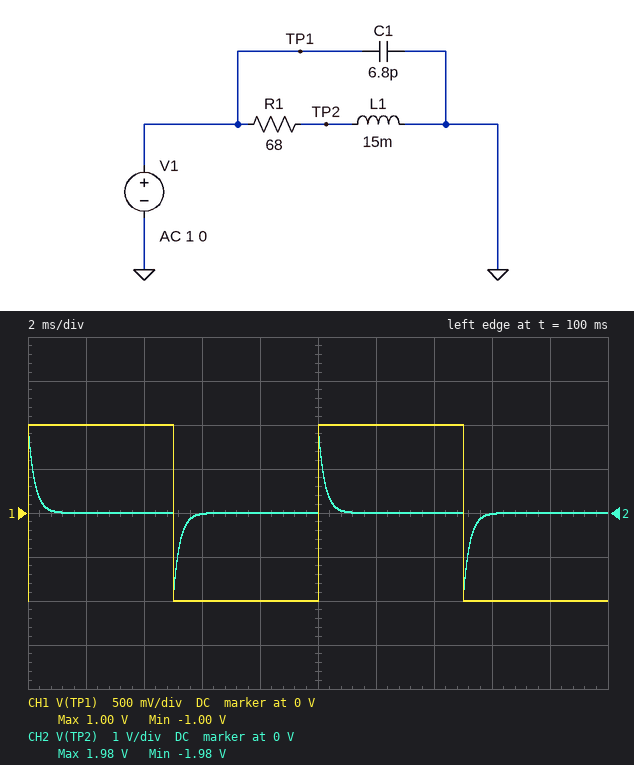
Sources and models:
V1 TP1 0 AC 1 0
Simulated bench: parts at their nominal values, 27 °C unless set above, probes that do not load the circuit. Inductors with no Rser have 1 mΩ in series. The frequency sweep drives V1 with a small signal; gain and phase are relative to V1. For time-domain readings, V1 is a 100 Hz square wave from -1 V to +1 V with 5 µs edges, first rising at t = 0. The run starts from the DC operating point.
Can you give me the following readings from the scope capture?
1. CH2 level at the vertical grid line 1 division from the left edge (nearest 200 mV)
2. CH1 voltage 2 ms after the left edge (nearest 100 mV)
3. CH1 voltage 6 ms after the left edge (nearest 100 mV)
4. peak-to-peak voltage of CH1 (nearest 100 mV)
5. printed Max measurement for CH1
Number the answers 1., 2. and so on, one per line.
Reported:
1. 0 V
2. 1.0 V
3. -1.0 V
4. 2.0 V
5. 1.00 V
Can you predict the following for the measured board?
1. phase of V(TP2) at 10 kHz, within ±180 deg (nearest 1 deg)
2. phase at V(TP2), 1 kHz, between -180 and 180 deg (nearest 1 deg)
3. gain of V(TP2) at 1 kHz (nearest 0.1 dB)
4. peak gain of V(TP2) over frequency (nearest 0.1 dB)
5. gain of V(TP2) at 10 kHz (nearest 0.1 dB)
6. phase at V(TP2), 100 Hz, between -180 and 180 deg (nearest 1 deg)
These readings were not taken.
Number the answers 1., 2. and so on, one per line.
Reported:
1. 4 deg
2. 36 deg
3. -1.8 dB
4. 0 dB
5. 0 dB
6. 82 deg
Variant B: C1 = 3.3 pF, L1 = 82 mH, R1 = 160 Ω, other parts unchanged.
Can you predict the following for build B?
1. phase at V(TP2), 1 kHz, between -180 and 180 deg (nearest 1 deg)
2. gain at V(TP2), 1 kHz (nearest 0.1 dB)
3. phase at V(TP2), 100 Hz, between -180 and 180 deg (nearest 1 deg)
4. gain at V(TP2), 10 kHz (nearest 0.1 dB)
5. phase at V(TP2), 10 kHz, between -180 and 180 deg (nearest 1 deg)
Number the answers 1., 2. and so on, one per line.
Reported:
1. 17 deg
2. -0.4 dB
3. 72 deg
4. 0 dB
5. 2 deg
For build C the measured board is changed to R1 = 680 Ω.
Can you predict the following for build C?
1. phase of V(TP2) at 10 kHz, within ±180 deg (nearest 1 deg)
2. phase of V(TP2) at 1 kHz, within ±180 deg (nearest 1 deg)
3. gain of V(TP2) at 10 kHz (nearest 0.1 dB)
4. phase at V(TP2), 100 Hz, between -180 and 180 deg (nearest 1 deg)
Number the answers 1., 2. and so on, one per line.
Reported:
1. 36 deg
2. 82 deg
3. -1.8 dB
4. 89 deg
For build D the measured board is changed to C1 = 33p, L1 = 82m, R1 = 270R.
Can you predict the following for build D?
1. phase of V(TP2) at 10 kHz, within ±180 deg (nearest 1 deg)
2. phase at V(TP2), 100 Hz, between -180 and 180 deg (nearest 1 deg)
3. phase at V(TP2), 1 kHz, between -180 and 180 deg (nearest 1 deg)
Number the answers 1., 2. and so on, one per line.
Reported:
1. 3 deg
2. 79 deg
3. 28 deg
